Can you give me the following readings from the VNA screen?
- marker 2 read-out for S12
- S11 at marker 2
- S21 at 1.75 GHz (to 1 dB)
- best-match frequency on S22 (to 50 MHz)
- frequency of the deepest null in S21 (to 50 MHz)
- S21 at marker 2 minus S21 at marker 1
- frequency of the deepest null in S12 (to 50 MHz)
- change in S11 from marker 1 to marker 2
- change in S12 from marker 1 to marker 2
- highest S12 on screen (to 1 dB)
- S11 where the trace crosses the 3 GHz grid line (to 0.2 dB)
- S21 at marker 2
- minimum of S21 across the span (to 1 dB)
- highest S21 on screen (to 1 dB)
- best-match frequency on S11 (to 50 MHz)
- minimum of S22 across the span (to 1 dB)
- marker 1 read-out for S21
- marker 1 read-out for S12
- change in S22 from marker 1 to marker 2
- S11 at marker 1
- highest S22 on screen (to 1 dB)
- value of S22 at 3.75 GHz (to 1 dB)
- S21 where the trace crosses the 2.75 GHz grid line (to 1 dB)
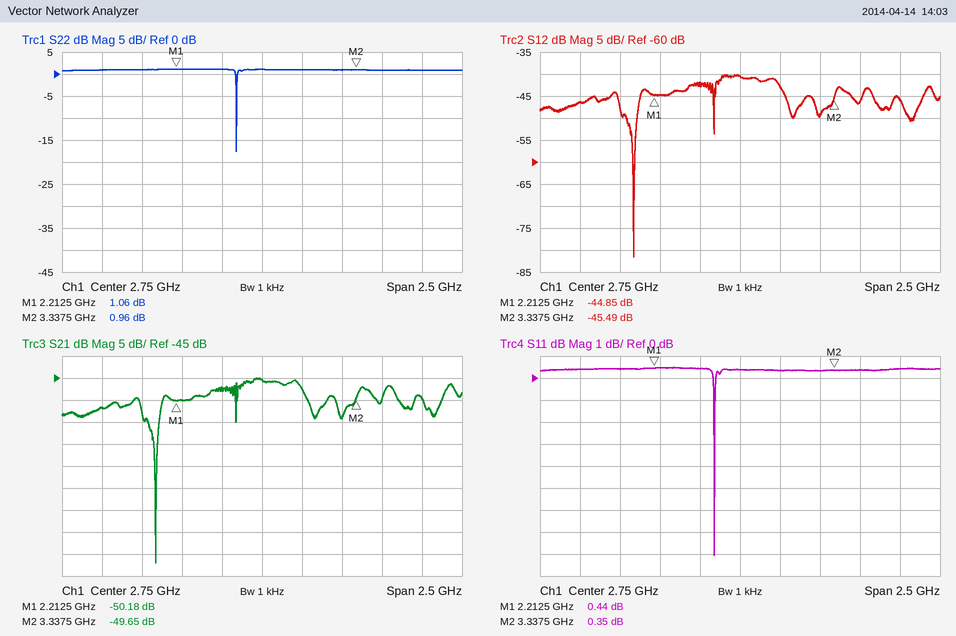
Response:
-45.49 dB
0.35 dB
-52 dB
2.60 GHz
2.10 GHz
0.53 dB
2.10 GHz
-0.09 dB
-0.64 dB
-40 dB
0.4 dB
-49.65 dB
-87 dB
-45 dB
2.60 GHz
-18 dB
-50.18 dB
-44.85 dB
-0.10 dB
0.44 dB
1 dB
1 dB
-45 dB
